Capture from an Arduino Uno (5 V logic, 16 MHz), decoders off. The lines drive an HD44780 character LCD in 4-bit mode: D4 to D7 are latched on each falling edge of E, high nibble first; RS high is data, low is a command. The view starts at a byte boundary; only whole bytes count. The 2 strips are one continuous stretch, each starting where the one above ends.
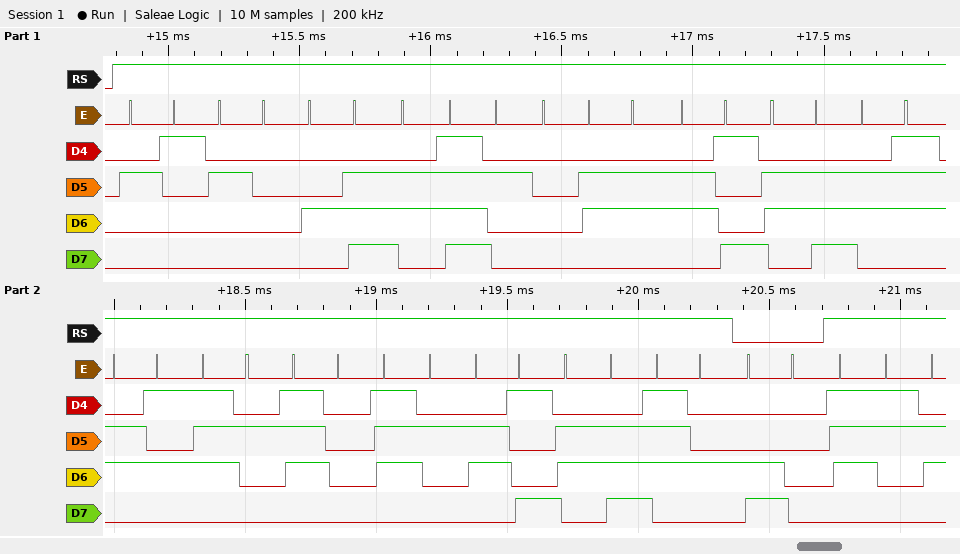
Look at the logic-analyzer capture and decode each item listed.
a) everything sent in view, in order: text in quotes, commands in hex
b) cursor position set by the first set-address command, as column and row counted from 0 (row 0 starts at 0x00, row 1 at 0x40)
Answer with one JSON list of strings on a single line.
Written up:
["\"! No fingerprint\" 0xC0 \"s\"", "column 0, row 1"]
